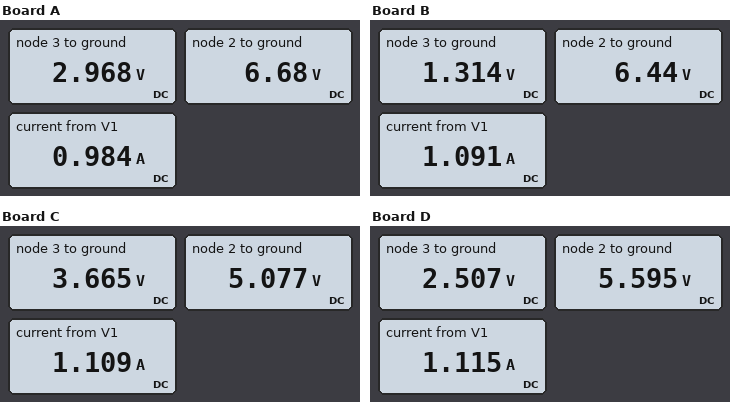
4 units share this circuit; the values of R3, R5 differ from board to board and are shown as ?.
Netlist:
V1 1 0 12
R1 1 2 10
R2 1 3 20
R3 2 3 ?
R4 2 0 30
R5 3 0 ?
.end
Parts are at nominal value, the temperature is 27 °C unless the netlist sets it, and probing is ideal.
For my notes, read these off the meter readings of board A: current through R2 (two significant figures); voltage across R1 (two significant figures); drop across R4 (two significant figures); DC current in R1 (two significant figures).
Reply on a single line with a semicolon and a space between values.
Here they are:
450 mA; 5.3 V; 6.7 V; 530 mA
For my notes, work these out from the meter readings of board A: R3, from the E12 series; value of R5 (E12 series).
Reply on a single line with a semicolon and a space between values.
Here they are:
12 Ω; 3.9 Ω
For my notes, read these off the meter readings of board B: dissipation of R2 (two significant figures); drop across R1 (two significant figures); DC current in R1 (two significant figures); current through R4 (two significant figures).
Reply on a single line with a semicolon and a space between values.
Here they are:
5.7 W; 5.6 V; 560 mA; 210 mA
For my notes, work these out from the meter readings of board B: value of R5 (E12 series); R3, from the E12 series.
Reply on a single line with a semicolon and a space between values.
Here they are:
1.5 Ω; 15 Ω
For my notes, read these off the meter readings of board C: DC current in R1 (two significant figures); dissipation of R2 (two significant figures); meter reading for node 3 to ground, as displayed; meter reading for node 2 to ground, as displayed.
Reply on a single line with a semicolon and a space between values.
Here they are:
690 mA; 3.5 W; 3.665 V; 5.077 V
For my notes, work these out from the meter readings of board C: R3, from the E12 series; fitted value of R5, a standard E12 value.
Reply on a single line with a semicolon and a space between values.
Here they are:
2.7 Ω; 3.9 Ω
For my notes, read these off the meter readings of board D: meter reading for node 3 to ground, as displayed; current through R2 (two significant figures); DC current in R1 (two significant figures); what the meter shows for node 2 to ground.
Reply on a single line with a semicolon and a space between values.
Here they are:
2.507 V; 470 mA; 640 mA; 5.595 V
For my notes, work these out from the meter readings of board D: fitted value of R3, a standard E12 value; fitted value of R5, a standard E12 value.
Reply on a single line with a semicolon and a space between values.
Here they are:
6.8 Ω; 2.7 Ω
